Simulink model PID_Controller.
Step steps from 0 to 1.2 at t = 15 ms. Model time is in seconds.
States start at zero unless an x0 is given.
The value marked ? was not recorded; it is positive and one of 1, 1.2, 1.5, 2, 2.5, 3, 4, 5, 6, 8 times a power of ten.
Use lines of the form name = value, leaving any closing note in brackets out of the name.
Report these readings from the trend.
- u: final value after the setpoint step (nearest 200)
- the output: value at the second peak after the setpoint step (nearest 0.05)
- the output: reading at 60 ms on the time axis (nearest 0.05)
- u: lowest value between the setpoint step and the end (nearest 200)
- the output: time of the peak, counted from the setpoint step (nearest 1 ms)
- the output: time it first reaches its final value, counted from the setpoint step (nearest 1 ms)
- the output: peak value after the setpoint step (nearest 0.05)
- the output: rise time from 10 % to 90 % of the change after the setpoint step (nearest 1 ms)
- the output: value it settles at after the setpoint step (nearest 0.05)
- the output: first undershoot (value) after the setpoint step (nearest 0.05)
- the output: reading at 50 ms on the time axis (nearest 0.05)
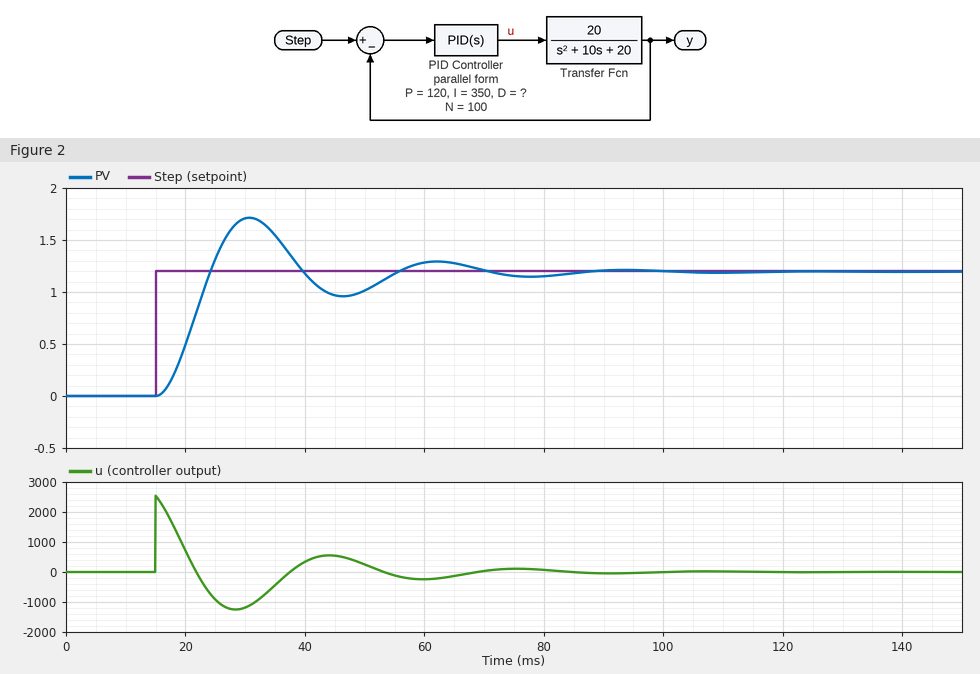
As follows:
u: final value after the setpoint step = 0
the output: value at the second peak after the setpoint step = 1.30
the output: reading at 60 ms on the time axis = 1.30
u: lowest value between the setpoint step and the end = -1200
the output: time of the peak, counted from the setpoint step = 16 ms
the output: time it first reaches its final value, counted from the setpoint step = 9 ms
the output: peak value after the setpoint step = 1.70
the output: rise time from 10 % to 90 % of the change after the setpoint step = 6 ms
the output: value it settles at after the setpoint step = 1.20
the output: first undershoot (value) after the setpoint step = 0.95
the output: reading at 50 ms on the time axis = 1.00
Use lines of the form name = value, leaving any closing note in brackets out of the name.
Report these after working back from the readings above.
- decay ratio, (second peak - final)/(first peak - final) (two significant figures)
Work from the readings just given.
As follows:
decay ratio, (second peak - final)/(first peak - final) = 0.20
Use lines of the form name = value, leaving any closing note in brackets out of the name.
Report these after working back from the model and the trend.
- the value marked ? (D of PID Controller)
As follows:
the value marked ? = 20
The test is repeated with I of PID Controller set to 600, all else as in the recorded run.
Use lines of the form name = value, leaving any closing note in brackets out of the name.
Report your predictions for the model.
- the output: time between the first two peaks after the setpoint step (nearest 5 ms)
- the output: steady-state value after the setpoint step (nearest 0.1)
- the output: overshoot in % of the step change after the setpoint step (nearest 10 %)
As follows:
the output: time between the first two peaks after the setpoint step = 30 ms
the output: steady-state value after the setpoint step = 1.2
the output: overshoot in % of the step change after the setpoint step = 40 %
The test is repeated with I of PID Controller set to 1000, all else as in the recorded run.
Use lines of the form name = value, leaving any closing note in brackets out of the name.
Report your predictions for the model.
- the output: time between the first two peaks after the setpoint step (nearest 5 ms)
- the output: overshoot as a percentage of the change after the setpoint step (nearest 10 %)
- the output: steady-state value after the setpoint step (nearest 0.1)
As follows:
the output: time between the first two peaks after the setpoint step = 30 ms
the output: overshoot as a percentage of the change after the setpoint step = 40 %
the output: steady-state value after the setpoint step = 1.2
